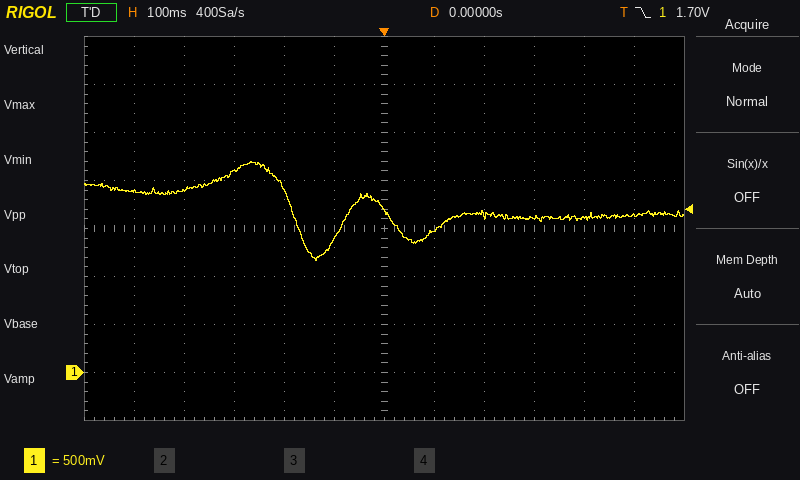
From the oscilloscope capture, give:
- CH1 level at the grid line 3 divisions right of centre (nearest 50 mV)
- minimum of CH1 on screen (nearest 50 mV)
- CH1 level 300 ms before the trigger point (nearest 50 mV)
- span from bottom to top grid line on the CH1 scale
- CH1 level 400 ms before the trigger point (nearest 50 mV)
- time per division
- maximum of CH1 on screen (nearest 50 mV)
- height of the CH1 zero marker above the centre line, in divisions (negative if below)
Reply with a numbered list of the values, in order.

1. 1.60 V
2. 1.15 V
3. 2.10 V
4. 4 V
5. 1.90 V
6. 100 ms
7. 2.20 V
8. -3.0 div
